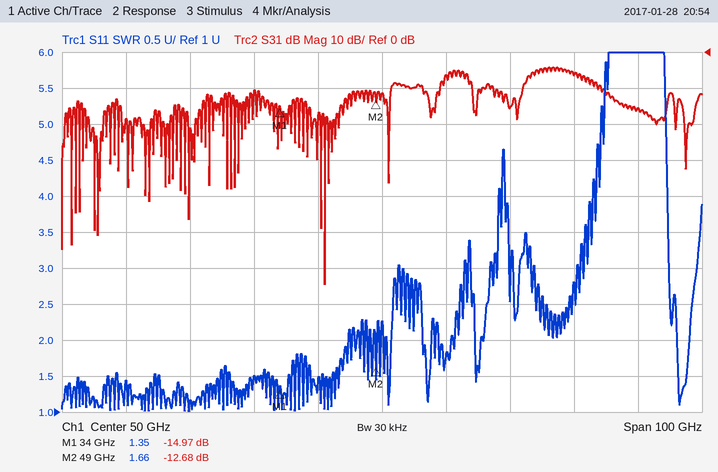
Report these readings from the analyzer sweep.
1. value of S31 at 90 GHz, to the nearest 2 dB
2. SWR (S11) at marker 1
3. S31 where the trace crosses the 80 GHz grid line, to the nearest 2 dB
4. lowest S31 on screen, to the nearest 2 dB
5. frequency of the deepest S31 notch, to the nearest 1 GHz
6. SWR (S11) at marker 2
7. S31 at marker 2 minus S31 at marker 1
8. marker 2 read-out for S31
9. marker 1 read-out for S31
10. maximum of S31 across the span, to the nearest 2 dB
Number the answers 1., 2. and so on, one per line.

1. -16 dB
2. 1.35
3. -6 dB
4. -64 dB
5. 41 GHz
6. 1.66
7. 2.29 dB
8. -12.68 dB
9. -14.97 dB
10. -4 dB
